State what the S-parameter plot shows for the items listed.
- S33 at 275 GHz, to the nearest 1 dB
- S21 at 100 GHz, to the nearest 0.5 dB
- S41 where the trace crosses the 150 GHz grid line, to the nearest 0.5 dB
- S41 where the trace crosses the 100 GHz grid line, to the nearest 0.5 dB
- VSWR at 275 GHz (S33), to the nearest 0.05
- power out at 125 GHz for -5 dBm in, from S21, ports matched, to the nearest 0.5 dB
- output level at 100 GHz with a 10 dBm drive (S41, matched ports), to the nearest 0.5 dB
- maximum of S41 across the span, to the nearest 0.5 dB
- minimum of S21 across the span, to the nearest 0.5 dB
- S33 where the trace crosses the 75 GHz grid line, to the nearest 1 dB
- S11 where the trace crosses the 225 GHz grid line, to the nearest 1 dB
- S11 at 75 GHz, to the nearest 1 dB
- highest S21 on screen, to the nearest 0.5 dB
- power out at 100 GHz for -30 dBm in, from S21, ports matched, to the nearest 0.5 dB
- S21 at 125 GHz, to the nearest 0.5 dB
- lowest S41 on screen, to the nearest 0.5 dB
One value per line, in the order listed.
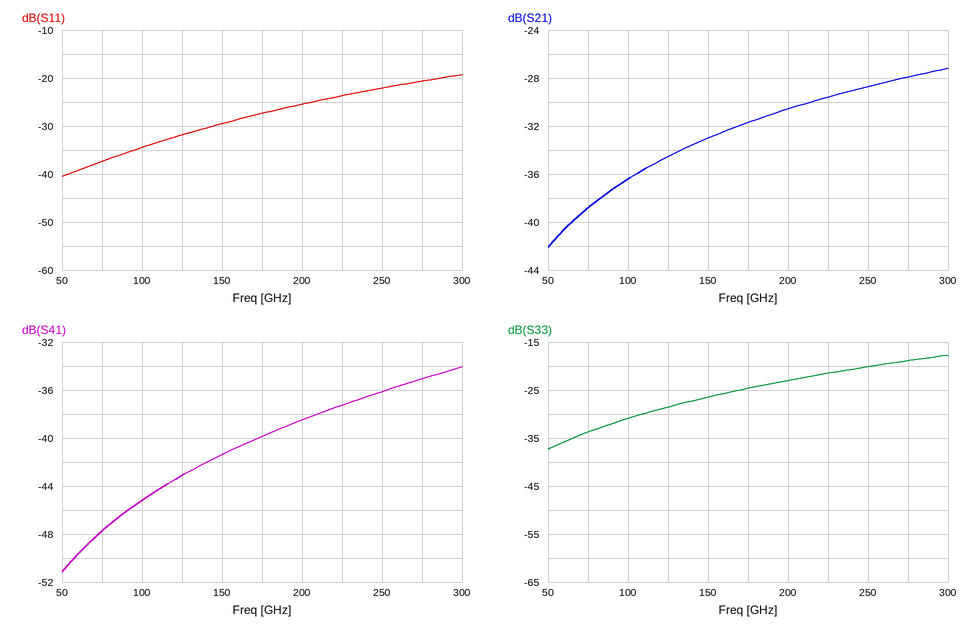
-19 dB
-36.5 dB
-41.5 dB
-45.0 dB
1.25
-39.5 dBm
-35.0 dBm
-34.0 dB
-42.0 dB
-34 dB
-24 dB
-37 dB
-27.0 dB
-66.5 dBm
-34.5 dB
-51.0 dB
